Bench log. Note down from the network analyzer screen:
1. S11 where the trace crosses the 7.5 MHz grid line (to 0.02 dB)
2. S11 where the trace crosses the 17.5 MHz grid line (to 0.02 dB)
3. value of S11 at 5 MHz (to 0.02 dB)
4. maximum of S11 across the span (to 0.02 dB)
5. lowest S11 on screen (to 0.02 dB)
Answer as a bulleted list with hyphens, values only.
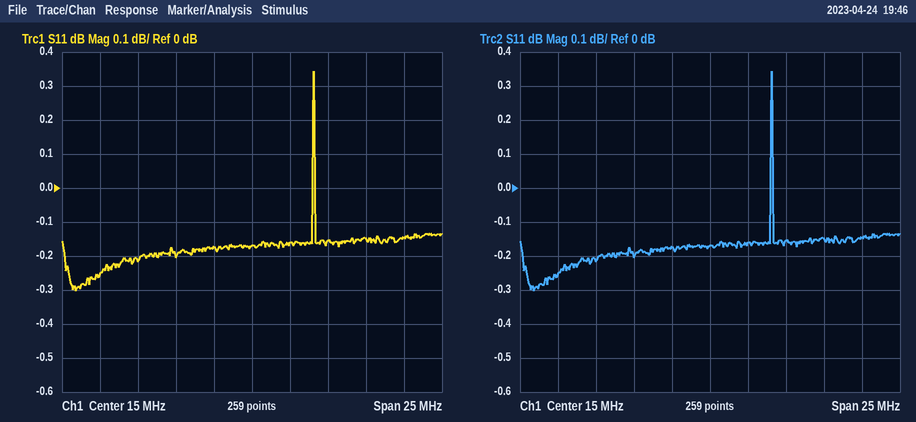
- -0.22 dB
- -0.16 dB
- -0.26 dB
- 0.34 dB
- -0.30 dB
